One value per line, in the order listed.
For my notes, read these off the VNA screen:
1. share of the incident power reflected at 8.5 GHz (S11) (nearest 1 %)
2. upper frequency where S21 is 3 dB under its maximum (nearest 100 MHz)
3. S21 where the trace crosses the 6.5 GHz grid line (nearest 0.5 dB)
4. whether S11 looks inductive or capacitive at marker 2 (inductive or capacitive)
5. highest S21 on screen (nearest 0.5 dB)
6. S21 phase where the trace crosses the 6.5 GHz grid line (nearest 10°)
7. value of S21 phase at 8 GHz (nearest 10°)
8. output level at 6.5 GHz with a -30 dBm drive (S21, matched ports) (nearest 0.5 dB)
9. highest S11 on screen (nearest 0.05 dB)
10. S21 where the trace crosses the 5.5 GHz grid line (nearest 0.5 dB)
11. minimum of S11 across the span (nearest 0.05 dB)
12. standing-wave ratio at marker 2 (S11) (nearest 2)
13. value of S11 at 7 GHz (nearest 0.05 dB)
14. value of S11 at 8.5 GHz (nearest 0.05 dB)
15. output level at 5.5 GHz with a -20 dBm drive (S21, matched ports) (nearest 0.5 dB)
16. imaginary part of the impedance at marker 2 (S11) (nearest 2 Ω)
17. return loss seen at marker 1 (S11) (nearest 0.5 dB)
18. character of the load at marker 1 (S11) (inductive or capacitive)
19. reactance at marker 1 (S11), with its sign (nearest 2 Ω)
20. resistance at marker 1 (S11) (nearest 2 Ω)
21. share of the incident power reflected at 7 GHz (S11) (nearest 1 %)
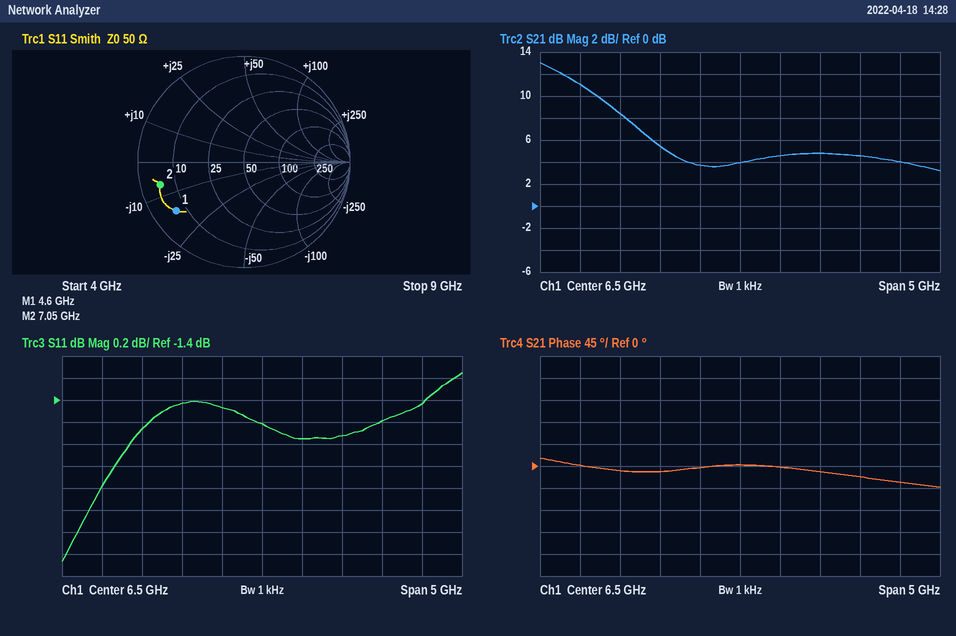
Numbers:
72 %
4.7 GHz
4.0 dB
capacitive
13.0 dB
0°
-20°
-26.0 dBm
-1.15 dB
5.5 dB
-2.85 dB
10
-1.75 dB
-1.45 dB
-14.5 dBm
-6 Ω
2.0 dB
capacitive
-16 Ω
6 Ω
67 %
